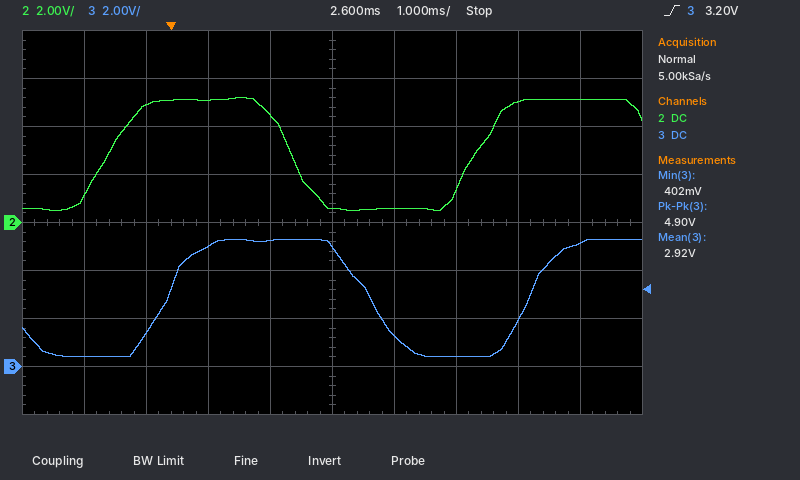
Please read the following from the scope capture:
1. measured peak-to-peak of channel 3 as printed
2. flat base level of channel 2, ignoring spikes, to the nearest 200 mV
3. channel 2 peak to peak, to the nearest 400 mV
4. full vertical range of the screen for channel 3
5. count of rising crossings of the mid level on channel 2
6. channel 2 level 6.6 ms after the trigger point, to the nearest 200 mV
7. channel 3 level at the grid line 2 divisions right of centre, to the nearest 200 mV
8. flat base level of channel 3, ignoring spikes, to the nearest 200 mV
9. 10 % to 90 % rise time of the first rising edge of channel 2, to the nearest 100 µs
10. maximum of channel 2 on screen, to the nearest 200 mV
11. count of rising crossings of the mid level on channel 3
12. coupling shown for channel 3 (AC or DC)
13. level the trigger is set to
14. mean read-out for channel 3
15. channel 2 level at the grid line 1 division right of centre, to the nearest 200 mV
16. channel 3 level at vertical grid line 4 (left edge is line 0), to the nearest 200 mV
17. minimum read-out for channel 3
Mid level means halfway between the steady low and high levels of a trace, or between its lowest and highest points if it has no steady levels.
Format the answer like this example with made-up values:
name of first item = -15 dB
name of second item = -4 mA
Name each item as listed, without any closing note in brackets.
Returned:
measured peak-to-peak of channel 3 as printed = 4.90 V
flat base level of channel 2, ignoring spikes, to the nearest 200 mV = 600 mV
channel 2 peak to peak, to the nearest 400 mV = 4.8 V
full vertical range of the screen for channel 3 = 16 V
count of rising crossings of the mid level on channel 2 = 2
channel 2 level 6.6 ms after the trigger point, to the nearest 200 mV = 5.2 V
channel 3 level at the grid line 2 divisions right of centre, to the nearest 200 mV = 400 mV
flat base level of channel 3, ignoring spikes, to the nearest 200 mV = 400 mV
10 % to 90 % rise time of the first rising edge of channel 2, to the nearest 100 µs = 900 µs
maximum of channel 2 on screen, to the nearest 200 mV = 5.2 V
count of rising crossings of the mid level on channel 3 = 2
coupling shown for channel 3 = DC
level the trigger is set to = 3.20 V
mean read-out for channel 3 = 2.92 V
channel 2 level at the grid line 1 division right of centre, to the nearest 200 mV = 600 mV
channel 3 level at vertical grid line 4 (left edge is line 0), to the nearest 200 mV = 5.2 V
minimum read-out for channel 3 = 402 mV
